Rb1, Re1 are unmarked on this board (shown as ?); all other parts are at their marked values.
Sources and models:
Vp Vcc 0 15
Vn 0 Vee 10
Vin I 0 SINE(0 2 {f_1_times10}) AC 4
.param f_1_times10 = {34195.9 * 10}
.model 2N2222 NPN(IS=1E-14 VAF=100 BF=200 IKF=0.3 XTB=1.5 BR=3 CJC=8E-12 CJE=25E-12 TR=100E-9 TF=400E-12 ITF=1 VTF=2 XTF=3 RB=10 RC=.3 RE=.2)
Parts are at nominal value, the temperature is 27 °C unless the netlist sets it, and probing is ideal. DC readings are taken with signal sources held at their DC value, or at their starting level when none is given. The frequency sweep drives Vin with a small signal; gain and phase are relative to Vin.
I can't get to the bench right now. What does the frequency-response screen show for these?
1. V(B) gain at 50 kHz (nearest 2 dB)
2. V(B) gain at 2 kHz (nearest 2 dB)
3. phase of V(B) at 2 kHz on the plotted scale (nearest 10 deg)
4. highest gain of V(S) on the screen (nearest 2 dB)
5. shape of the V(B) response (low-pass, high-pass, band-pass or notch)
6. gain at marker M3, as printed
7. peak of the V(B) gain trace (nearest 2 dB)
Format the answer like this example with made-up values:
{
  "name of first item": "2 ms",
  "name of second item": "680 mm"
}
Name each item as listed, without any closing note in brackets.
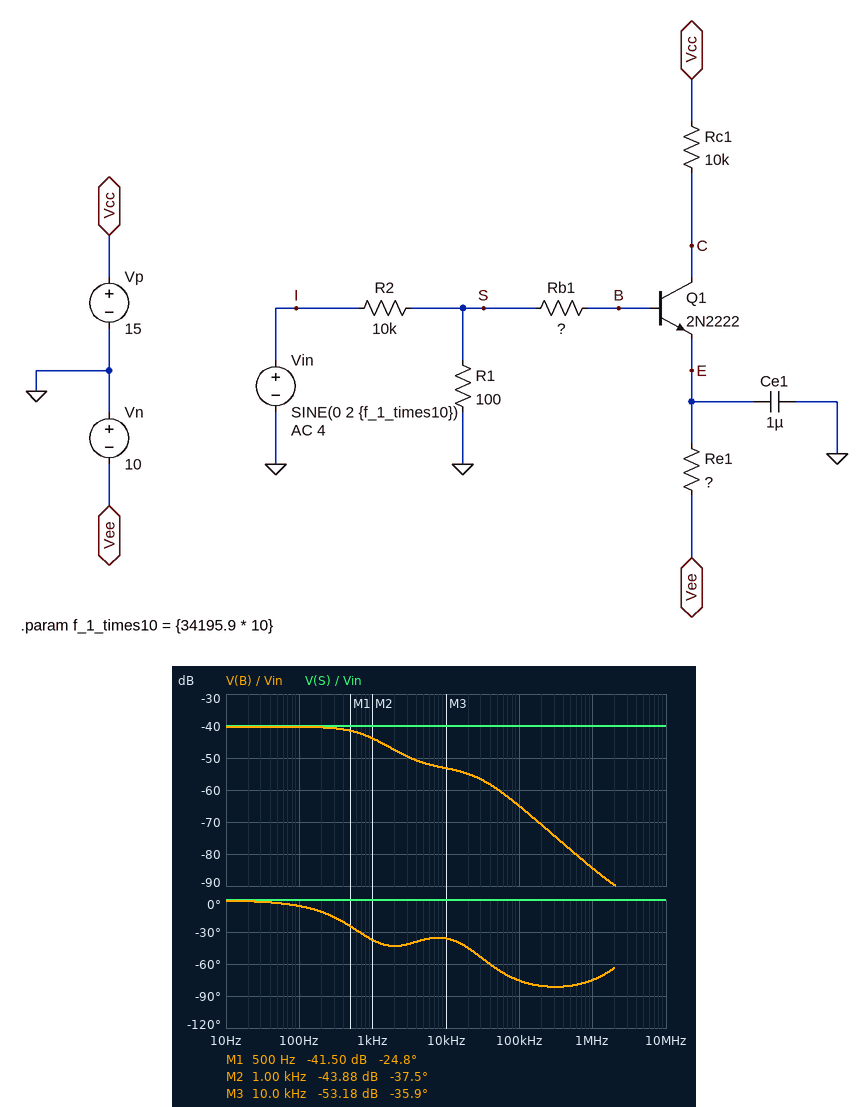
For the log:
{
  "V(B) gain at 50 kHz": "-60 dB",
  "V(B) gain at 2 kHz": "-48 dB",
  "phase of V(B) at 2 kHz on the plotted scale": "-40 deg",
  "highest gain of V(S) on the screen": "-40 dB",
  "shape of the V(B) response": "low-pass",
  "gain at marker M3, as printed": "-53.18 dB",
  "peak of the V(B) gain trace": "-40 dB"
}
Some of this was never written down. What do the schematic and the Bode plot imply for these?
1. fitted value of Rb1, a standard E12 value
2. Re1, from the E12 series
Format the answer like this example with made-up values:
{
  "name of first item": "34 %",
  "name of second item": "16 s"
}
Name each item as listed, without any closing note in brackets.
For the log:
{
  "fitted value of Rb1, a standard E12 value": "33 kΩ",
  "Re1, from the E12 series": "15 kΩ"
}
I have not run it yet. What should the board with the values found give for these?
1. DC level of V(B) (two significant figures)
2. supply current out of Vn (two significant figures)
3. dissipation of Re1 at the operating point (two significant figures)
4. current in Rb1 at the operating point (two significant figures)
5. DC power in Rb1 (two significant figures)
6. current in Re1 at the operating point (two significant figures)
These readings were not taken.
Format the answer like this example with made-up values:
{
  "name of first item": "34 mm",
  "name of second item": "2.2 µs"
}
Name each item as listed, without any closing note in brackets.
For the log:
{
  "DC level of V(B)": "-94 mV",
  "supply current out of Vn": "620 µA",
  "dissipation of Re1 at the operating point": "5.7 mW",
  "current in Rb1 at the operating point": "2.8 µA",
  "DC power in Rb1": "260 nW",
  "current in Re1 at the operating point": "620 µA"
}
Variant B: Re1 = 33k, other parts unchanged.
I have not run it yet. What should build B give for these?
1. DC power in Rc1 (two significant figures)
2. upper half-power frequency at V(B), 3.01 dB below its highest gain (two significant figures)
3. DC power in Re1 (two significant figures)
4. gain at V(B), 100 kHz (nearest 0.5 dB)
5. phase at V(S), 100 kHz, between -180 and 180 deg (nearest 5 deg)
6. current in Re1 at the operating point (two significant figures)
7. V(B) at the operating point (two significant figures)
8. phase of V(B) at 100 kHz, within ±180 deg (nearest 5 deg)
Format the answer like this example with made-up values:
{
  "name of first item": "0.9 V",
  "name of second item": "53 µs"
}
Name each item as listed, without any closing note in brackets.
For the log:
{
  "DC power in Rc1": "790 µW",
  "upper half-power frequency at V(B), 3.01 dB below its highest gain": "800 Hz",
  "DC power in Re1": "2.6 mW",
  "gain at V(B), 100 kHz": "-58.5 dB",
  "phase at V(S), 100 kHz, between -180 and 180 deg": "0 deg",
  "current in Re1 at the operating point": "280 µA",
  "V(B) at the operating point": "-42 mV",
  "phase of V(B) at 100 kHz, within ±180 deg": "-70 deg"
}
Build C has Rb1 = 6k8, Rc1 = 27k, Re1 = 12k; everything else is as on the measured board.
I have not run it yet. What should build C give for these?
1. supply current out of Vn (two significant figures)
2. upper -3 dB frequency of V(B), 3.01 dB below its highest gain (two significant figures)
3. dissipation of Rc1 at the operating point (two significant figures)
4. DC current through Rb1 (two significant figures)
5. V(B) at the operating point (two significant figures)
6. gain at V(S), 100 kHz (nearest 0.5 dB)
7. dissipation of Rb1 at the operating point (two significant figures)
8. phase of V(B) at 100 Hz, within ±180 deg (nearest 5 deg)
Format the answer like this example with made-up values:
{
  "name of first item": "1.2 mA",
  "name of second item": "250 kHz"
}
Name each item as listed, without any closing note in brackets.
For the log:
{
  "supply current out of Vn": "720 µA",
  "upper -3 dB frequency of V(B), 3.01 dB below its highest gain": "42 Hz",
  "dissipation of Rc1 at the operating point": "9.9 mW",
  "DC current through Rb1": "110 µA",
  "V(B) at the operating point": "-750 mV",
  "gain at V(S), 100 kHz": "-40.0 dB",
  "dissipation of Rb1 at the operating point": "81 µW",
  "phase of V(B) at 100 Hz, within ±180 deg": "-65 deg"
}
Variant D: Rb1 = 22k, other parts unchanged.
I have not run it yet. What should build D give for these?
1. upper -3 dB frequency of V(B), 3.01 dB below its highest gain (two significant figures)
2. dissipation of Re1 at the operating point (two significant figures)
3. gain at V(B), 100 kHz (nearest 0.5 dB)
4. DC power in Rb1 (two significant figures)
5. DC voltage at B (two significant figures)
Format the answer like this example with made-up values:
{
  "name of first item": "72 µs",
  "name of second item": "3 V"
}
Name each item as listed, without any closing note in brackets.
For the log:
{
  "upper -3 dB frequency of V(B), 3.01 dB below its highest gain": "1.2 kHz",
  "dissipation of Re1 at the operating point": "5.8 mW",
  "gain at V(B), 100 kHz": "-61.5 dB",
  "DC power in Rb1": "180 nW",
  "DC voltage at B": "-63 mV"
}
